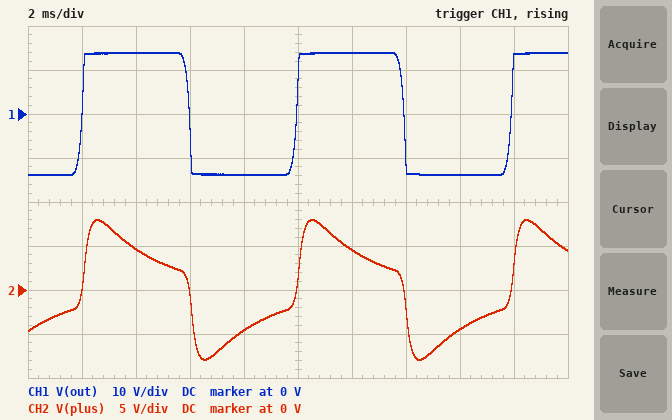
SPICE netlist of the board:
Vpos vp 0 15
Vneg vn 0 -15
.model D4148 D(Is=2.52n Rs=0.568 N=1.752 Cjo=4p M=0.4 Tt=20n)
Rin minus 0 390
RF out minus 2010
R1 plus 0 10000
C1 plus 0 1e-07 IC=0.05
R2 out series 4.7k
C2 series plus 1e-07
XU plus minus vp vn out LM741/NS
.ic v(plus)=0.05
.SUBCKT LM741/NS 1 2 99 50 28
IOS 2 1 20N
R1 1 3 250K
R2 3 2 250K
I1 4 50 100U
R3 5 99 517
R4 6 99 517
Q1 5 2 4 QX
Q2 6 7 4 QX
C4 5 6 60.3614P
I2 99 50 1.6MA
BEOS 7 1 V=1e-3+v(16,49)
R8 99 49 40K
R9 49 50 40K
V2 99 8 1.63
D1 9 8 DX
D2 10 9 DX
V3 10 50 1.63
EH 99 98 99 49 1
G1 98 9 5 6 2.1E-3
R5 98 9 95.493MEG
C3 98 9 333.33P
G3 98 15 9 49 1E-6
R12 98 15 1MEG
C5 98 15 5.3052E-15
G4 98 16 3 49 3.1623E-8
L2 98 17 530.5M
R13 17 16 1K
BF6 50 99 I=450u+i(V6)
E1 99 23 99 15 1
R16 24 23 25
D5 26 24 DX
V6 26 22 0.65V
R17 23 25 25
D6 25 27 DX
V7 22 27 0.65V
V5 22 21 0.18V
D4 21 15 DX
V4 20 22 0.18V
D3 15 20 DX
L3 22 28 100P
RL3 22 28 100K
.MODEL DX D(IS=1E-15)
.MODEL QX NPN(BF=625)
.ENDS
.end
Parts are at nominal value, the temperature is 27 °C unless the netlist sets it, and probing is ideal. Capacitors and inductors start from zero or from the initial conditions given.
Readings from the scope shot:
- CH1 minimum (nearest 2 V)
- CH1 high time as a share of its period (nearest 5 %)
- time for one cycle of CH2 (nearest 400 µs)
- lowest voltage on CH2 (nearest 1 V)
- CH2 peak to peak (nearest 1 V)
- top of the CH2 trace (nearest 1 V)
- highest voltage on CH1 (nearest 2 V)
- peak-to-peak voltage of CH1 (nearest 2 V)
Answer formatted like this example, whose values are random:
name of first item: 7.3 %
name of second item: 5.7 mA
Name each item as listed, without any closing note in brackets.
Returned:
CH1 minimum: -14 V
CH1 high time as a share of its period: 50 %
time for one cycle of CH2: 8.0 ms
lowest voltage on CH2: -8 V
CH2 peak to peak: 16 V
top of the CH2 trace: 8 V
highest voltage on CH1: 14 V
peak-to-peak voltage of CH1: 28 V
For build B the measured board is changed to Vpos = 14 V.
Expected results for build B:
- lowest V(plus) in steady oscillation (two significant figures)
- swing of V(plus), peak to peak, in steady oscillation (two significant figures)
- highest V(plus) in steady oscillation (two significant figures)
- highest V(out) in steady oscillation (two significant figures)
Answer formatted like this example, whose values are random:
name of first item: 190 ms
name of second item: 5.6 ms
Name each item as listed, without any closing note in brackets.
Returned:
lowest V(plus) in steady oscillation: -7.7 V
swing of V(plus), peak to peak, in steady oscillation: 15 V
highest V(plus) in steady oscillation: 7.6 V
highest V(out) in steady oscillation: 13 V
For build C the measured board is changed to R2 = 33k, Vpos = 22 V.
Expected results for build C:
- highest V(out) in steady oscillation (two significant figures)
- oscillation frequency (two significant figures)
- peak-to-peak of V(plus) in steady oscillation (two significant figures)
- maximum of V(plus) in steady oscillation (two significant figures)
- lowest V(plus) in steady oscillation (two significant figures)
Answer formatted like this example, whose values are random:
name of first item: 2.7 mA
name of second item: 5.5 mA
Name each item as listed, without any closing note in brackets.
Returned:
highest V(out) in steady oscillation: 21 V
oscillation frequency: 81 Hz
peak-to-peak of V(plus) in steady oscillation: 7.4 V
maximum of V(plus) in steady oscillation: 3.9 V
lowest V(plus) in steady oscillation: -3.4 V
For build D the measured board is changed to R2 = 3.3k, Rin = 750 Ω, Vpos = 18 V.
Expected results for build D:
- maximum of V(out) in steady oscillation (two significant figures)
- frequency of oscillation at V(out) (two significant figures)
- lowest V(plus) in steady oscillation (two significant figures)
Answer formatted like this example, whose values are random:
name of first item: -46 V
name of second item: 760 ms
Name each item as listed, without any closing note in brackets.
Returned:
maximum of V(out) in steady oscillation: 17 V
frequency of oscillation at V(out): 190 Hz
lowest V(plus) in steady oscillation: -8.2 V
